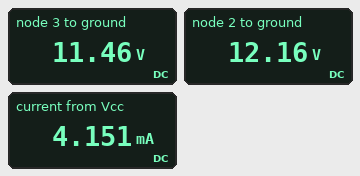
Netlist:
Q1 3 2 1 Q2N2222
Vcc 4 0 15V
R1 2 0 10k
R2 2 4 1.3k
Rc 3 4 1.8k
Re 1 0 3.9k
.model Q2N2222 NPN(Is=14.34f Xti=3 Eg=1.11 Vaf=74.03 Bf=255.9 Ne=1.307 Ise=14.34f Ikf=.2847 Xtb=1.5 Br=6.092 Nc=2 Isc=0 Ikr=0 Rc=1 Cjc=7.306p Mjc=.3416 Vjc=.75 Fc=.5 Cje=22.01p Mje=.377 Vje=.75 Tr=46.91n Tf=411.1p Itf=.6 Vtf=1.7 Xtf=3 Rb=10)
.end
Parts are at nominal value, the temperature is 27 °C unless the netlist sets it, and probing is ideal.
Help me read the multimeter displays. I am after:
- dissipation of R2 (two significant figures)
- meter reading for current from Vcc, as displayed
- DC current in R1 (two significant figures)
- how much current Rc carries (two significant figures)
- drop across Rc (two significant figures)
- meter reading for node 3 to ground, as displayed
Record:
6.2 mW
4.151 mA
1.2 mA
2.0 mA
3.5 V
11.46 V
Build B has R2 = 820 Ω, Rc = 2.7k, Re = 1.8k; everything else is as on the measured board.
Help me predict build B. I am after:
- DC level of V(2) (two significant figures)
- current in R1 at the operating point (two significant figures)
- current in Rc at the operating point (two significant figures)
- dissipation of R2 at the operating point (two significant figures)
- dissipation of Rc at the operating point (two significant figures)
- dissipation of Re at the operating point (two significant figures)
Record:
11 V
1.1 mA
1.8 mA
20 mW
8.6 mW
57 mW
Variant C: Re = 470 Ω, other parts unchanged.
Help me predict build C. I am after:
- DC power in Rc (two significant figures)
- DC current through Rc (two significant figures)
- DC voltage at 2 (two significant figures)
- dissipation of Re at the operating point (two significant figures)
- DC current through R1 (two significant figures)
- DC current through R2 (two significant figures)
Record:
51 mW
5.3 mA
6.2 V
62 mW
620 µA
6.8 mA
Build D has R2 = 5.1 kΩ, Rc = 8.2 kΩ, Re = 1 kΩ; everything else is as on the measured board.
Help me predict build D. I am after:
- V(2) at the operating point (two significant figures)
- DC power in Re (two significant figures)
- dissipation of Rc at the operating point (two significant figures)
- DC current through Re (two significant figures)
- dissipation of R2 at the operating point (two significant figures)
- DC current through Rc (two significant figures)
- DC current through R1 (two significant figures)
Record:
3.9 V
10 mW
17 mW
3.2 mA
24 mW
1.4 mA
390 µA
